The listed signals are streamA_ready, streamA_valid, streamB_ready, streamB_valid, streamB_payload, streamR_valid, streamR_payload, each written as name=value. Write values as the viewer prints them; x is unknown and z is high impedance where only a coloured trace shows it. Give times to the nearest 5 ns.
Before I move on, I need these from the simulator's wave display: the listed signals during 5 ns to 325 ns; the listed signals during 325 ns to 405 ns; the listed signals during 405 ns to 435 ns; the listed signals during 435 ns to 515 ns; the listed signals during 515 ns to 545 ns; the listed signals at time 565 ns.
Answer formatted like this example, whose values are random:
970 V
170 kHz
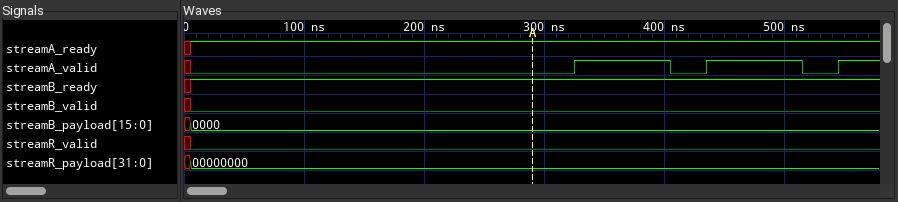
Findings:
streamA_ready=1, streamA_valid=0, streamB_ready=1, streamB_valid=0, streamB_payload=0000, streamR_valid=0, streamR_payload=00000000
streamA_ready=1, streamA_valid=1, streamB_ready=1, streamB_valid=0, streamB_payload=0000, streamR_valid=0, streamR_payload=00000000
streamA_ready=1, streamA_valid=0, streamB_ready=1, streamB_valid=0, streamB_payload=0000, streamR_valid=0, streamR_payload=00000000
streamA_ready=1, streamA_valid=1, streamB_ready=1, streamB_valid=0, streamB_payload=0000, streamR_valid=0, streamR_payload=00000000
streamA_ready=1, streamA_valid=0, streamB_ready=1, streamB_valid=0, streamB_payload=0000, streamR_valid=0, streamR_payload=00000000
streamA_ready=1, streamA_valid=1, streamB_ready=1, streamB_valid=0, streamB_payload=0000, streamR_valid=0, streamR_payload=00000000
